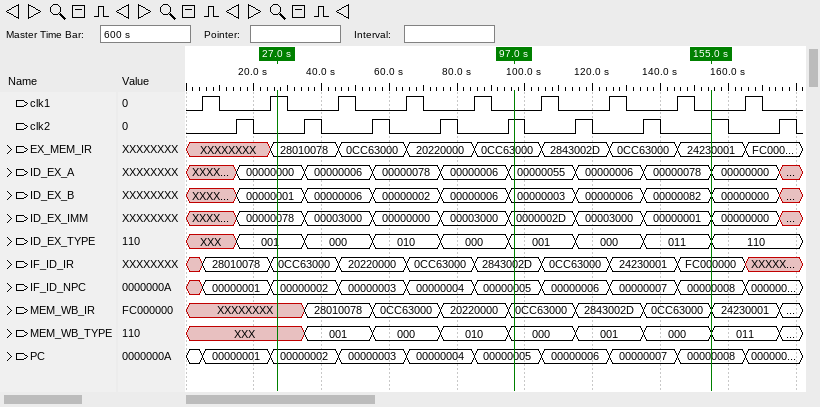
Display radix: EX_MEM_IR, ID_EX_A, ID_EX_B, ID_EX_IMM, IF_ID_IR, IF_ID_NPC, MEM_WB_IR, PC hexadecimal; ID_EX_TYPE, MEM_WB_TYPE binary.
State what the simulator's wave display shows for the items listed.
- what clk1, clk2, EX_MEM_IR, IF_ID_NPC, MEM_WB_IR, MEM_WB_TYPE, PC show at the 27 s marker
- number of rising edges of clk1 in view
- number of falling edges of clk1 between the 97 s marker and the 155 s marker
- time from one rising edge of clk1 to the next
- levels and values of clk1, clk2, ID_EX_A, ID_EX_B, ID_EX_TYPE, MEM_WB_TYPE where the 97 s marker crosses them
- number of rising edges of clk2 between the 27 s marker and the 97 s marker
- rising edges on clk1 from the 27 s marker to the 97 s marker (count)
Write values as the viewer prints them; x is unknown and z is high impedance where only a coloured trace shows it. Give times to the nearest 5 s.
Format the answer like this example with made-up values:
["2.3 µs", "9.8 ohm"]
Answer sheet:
["clk1=1, clk2=0, EX_MEM_IR=28010078, IF_ID_NPC=00000002, MEM_WB_IR=XXXXXXXX, MEM_WB_TYPE=XXX, PC=00000002", "9", "3", "20 s", "clk1=0, clk2=1, ID_EX_A=00000055, ID_EX_B=00000003, ID_EX_TYPE=001, MEM_WB_TYPE=000", "4", "3"]
